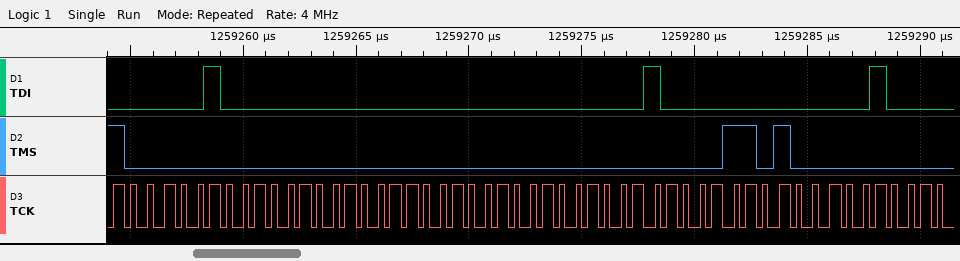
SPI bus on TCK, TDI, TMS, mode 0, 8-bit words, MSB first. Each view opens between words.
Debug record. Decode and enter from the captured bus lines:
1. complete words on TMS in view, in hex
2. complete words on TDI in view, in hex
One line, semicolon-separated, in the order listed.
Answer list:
80, 00, 00, 00, 00, D0; 02, 00, 00, 00, 10, 00
